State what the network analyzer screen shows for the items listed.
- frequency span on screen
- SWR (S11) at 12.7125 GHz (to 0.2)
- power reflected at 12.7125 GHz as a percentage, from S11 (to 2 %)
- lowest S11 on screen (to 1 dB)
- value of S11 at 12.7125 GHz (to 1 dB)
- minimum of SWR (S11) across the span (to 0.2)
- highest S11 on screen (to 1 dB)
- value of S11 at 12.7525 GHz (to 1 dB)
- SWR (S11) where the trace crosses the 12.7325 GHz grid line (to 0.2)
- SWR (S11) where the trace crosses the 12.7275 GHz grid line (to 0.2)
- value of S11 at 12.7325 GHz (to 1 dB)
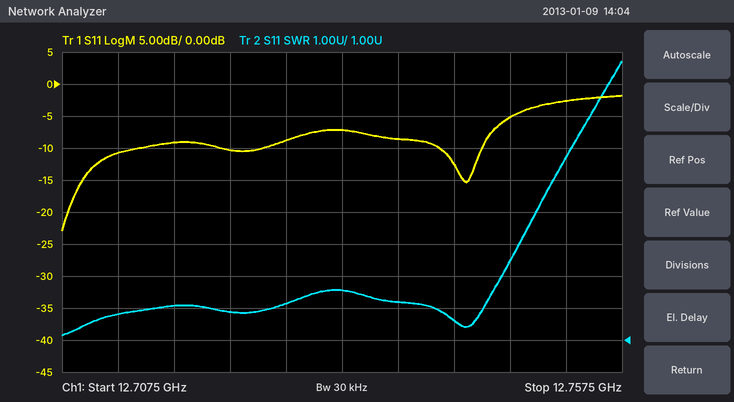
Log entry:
50 MHz
1.8
8 %
-23 dB
-11 dB
1.2
-2 dB
-3 dB
2.6
2.2
-7 dB
